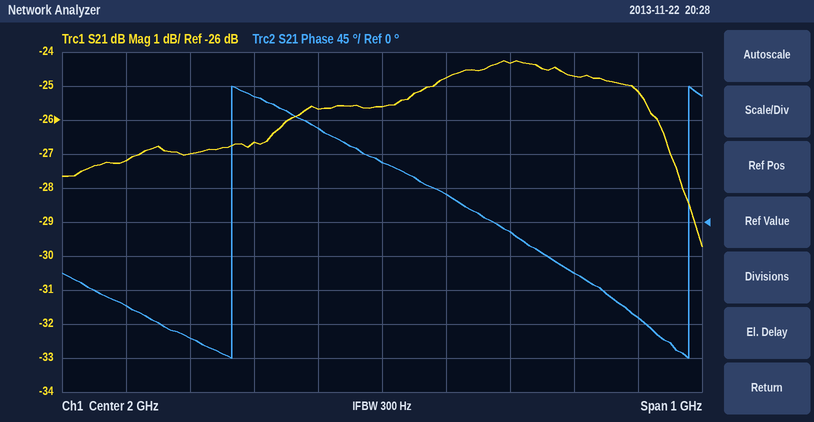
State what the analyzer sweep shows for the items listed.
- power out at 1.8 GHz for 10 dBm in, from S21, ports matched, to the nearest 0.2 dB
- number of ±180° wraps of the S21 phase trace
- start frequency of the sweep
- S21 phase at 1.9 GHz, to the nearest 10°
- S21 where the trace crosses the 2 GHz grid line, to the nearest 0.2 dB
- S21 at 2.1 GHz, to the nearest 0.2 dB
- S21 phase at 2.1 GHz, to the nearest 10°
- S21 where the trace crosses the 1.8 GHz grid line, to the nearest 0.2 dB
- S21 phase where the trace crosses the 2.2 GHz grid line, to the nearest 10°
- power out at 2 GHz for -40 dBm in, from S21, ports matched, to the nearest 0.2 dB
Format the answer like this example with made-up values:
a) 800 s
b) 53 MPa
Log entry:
a) -16.6 dBm
b) 2
c) 1.5 GHz
d) 120°
e) -25.6 dB
f) -24.8 dB
g) 40°
h) -26.6 dB
i) -10°
j) -65.6 dBm
